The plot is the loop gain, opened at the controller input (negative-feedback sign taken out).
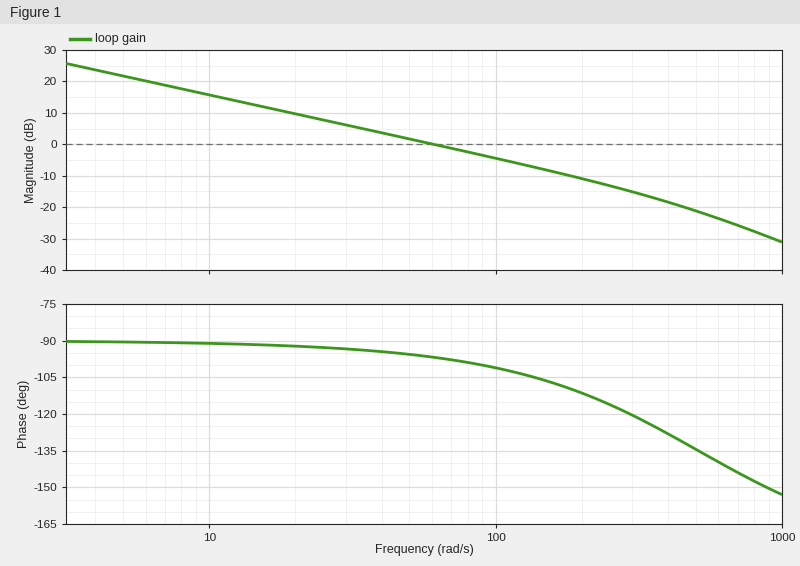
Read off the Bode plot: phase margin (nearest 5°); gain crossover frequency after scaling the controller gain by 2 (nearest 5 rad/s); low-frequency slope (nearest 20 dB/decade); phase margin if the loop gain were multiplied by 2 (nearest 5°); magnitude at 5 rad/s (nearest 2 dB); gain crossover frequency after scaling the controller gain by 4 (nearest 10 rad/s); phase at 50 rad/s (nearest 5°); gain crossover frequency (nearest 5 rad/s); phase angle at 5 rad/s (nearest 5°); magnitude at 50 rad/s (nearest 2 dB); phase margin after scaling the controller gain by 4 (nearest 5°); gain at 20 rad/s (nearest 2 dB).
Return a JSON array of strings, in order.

["85°", "120 rad/s", "-20 dB/decade", "75°", "22 dB", "220 rad/s", "-95°", "60 rad/s", "-90°", "2 dB", "65°", "10 dB"]
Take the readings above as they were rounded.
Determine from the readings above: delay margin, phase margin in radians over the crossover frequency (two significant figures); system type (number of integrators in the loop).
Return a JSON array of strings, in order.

["0.025 s", "1"]
